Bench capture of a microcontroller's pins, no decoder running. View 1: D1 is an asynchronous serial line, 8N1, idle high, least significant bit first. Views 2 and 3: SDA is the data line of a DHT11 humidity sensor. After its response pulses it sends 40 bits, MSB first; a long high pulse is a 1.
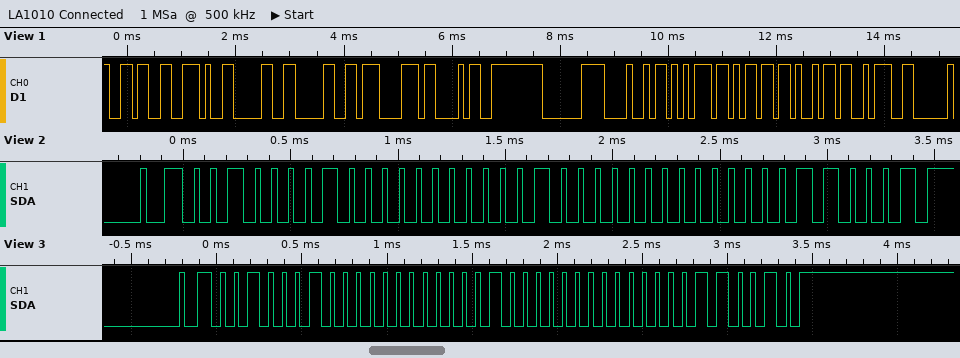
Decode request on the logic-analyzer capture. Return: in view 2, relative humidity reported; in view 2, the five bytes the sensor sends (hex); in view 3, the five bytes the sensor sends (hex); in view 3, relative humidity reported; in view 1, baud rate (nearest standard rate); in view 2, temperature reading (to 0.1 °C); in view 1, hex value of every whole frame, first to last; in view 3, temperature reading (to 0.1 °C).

33 %
21 00 10 00 31
22 00 10 00 32
34 %
9600 baud
16.0 °C
36 2E 30 30 87 43 FE C0 48 75 6D 69 3A
16.0 °C
